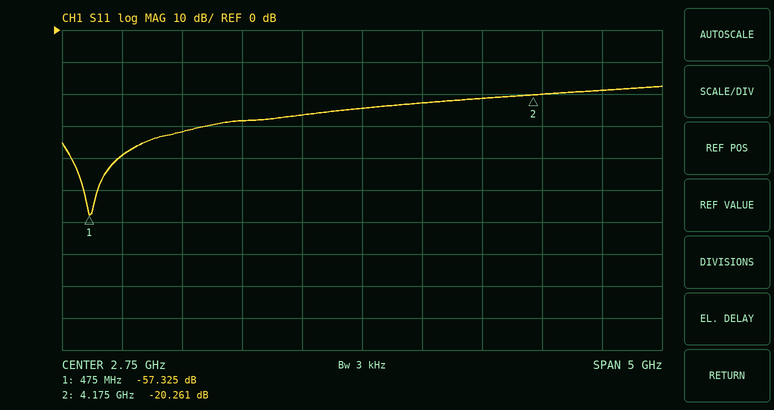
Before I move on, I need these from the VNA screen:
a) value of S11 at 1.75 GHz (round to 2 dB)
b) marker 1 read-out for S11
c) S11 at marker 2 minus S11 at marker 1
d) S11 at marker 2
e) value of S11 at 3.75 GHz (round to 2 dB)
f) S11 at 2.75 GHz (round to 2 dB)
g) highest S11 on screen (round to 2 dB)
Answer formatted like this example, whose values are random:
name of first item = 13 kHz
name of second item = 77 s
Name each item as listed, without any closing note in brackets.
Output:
value of S11 at 1.75 GHz = -28 dB
marker 1 read-out for S11 = -57.325 dB
S11 at marker 2 minus S11 at marker 1 = 37.064 dB
S11 at marker 2 = -20.261 dB
value of S11 at 3.75 GHz = -22 dB
S11 at 2.75 GHz = -24 dB
highest S11 on screen = -18 dB
